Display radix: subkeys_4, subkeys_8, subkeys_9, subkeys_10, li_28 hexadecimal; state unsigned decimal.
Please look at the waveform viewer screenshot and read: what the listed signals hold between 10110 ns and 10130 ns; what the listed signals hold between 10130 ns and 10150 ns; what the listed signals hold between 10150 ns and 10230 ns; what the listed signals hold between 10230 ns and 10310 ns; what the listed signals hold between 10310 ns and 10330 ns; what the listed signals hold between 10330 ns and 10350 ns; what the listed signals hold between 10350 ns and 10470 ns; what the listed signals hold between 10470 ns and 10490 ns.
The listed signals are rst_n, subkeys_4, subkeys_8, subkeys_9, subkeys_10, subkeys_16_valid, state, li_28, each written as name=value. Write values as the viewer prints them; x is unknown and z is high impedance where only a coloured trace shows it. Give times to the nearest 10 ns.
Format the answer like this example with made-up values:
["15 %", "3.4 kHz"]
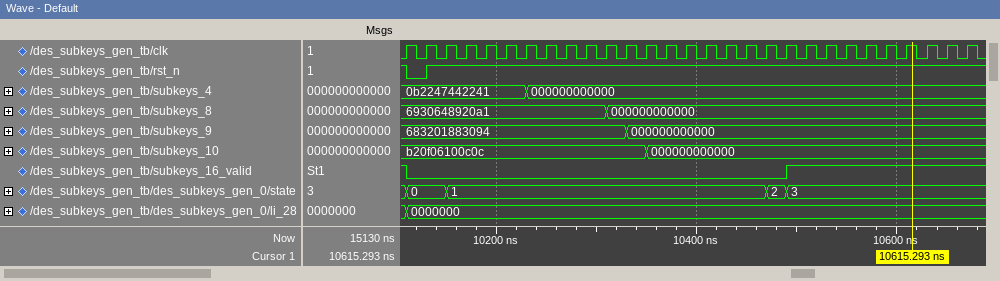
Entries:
["rst_n=0, subkeys_4=0b2247442241, subkeys_8=6930648920a1, subkeys_9=683201883094, subkeys_10=b20f06100c0c, subkeys_16_valid=0, state=0, li_28=0000000", "rst_n=1, subkeys_4=0b2247442241, subkeys_8=6930648920a1, subkeys_9=683201883094, subkeys_10=b20f06100c0c, subkeys_16_valid=0, state=0, li_28=0000000", "rst_n=1, subkeys_4=0b2247442241, subkeys_8=6930648920a1, subkeys_9=683201883094, subkeys_10=b20f06100c0c, subkeys_16_valid=0, state=1, li_28=0000000", "rst_n=1, subkeys_4=000000000000, subkeys_8=6930648920a1, subkeys_9=683201883094, subkeys_10=b20f06100c0c, subkeys_16_valid=0, state=1, li_28=0000000", "rst_n=1, subkeys_4=000000000000, subkeys_8=000000000000, subkeys_9=683201883094, subkeys_10=b20f06100c0c, subkeys_16_valid=0, state=1, li_28=0000000", "rst_n=1, subkeys_4=000000000000, subkeys_8=000000000000, subkeys_9=000000000000, subkeys_10=b20f06100c0c, subkeys_16_valid=0, state=1, li_28=0000000", "rst_n=1, subkeys_4=000000000000, subkeys_8=000000000000, subkeys_9=000000000000, subkeys_10=000000000000, subkeys_16_valid=0, state=1, li_28=0000000", "rst_n=1, subkeys_4=000000000000, subkeys_8=000000000000, subkeys_9=000000000000, subkeys_10=000000000000, subkeys_16_valid=0, state=2, li_28=0000000"]
